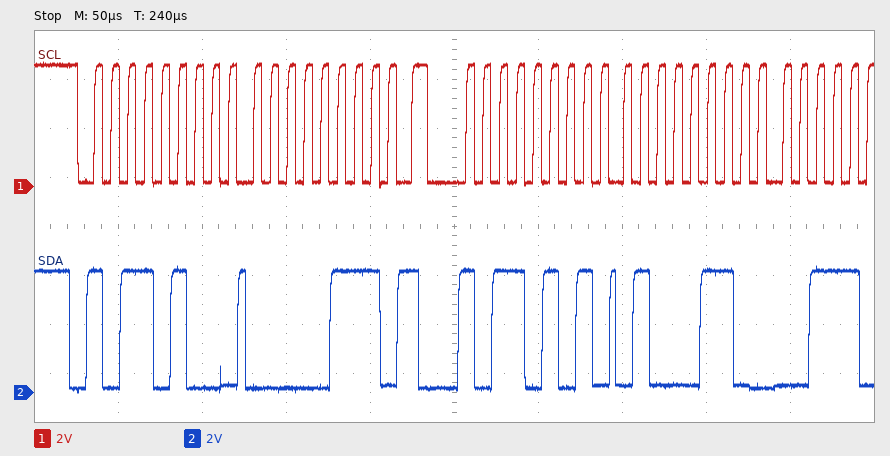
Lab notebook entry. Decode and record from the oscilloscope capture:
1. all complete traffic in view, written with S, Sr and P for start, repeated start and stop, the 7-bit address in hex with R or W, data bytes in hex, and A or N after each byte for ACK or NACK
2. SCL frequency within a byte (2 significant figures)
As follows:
S 5AW A 07 A Sr 5AR A 46 A
100 kHz
